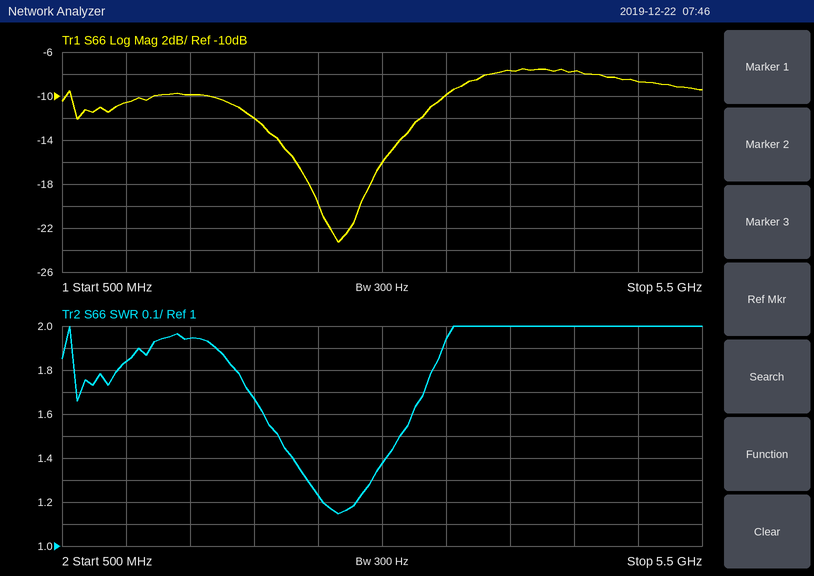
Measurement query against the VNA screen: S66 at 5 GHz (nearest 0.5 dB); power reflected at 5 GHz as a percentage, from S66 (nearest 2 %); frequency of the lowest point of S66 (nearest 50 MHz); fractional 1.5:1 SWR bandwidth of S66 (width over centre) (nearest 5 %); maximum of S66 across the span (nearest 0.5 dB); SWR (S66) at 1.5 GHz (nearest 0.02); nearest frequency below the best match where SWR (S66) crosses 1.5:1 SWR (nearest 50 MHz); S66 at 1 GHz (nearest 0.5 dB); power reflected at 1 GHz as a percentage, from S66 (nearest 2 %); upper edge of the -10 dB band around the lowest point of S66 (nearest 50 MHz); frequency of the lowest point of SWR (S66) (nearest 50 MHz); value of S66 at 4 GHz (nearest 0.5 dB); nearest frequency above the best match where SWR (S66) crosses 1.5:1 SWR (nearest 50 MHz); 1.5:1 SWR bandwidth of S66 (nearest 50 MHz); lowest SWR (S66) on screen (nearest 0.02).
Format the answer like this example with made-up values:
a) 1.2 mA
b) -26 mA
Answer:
a) -8.5 dB
b) 14 %
c) 2.65 GHz
d) 35 %
e) -7.5 dB
f) 1.94
g) 2.20 GHz
h) -10.5 dB
i) 8 %
j) 3.50 GHz
k) 2.65 GHz
l) -7.5 dB
m) 3.15 GHz
n) 950 MHz
o) 1.14
